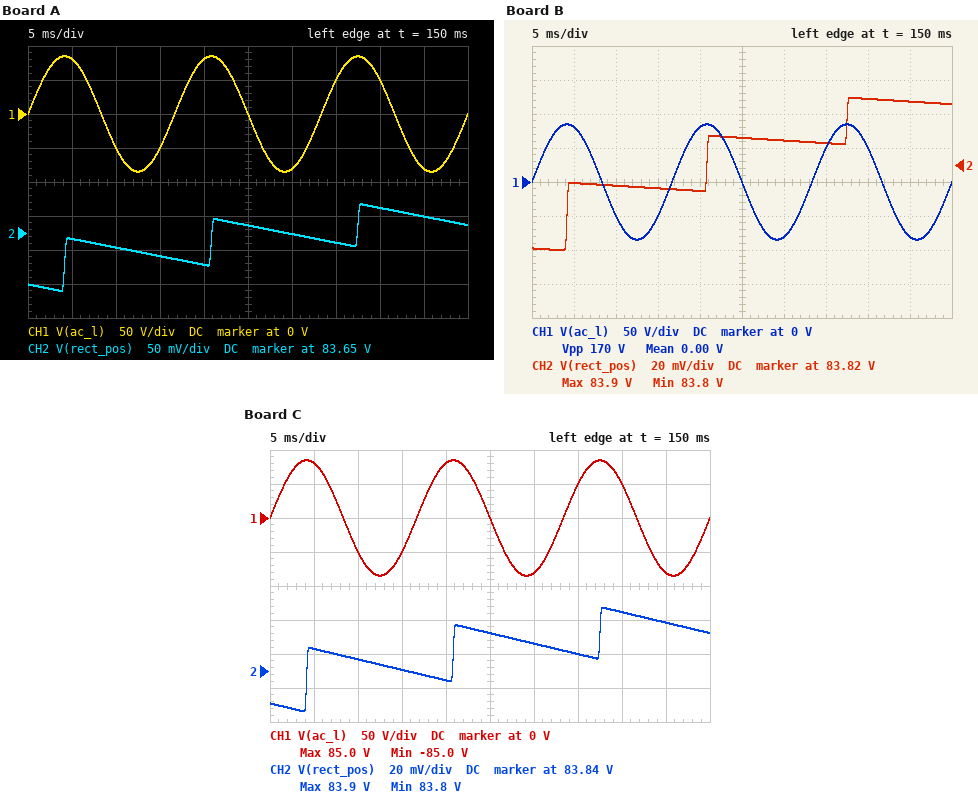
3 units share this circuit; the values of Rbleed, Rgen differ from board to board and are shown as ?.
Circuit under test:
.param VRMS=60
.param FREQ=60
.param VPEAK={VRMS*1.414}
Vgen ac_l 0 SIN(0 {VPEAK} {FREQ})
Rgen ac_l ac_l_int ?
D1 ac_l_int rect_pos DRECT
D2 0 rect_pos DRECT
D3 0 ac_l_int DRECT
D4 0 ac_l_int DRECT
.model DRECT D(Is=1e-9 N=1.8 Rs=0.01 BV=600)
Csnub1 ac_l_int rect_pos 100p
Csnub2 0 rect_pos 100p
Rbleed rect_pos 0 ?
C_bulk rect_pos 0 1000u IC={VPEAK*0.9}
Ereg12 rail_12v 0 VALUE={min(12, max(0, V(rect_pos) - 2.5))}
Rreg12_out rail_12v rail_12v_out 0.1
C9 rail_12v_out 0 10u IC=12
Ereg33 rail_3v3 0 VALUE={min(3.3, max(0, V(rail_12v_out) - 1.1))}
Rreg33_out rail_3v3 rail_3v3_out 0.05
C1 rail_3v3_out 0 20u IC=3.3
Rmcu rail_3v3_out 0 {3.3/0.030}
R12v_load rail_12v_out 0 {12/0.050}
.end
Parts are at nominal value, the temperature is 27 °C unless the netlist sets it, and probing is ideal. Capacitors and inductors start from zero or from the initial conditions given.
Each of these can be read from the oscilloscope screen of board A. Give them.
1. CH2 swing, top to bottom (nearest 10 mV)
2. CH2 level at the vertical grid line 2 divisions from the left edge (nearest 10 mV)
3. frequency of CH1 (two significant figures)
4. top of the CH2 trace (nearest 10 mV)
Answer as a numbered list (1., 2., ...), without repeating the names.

1. 130 mV
2. 83.63 V
3. 60 Hz
4. 83.69 V
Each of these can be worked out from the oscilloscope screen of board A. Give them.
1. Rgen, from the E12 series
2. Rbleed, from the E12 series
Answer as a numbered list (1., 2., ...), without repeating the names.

1. 1.5 Ω
2. 33 kΩ
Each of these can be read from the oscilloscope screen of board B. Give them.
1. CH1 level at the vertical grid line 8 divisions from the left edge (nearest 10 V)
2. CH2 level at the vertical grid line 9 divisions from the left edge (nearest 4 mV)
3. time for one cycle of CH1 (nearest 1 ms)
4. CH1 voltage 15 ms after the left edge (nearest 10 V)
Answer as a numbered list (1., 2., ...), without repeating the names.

1. 50 V
2. 83.856 V
3. 17 ms
4. -50 V
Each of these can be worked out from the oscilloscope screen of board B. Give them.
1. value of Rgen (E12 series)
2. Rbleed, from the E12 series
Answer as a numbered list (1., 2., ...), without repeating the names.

1. 1.2 Ω
2. 270 kΩ
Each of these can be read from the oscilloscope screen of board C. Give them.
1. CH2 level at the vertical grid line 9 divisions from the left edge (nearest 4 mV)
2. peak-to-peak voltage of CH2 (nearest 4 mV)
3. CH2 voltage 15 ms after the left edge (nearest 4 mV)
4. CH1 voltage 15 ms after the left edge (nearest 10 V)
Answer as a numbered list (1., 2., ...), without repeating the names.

1. 83.868 V
2. 60 mV
3. 83.840 V
4. -50 V
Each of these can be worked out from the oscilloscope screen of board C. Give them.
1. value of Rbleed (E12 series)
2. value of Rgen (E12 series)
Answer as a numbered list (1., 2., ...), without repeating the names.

1. 68 kΩ
2. 0.82 Ω
